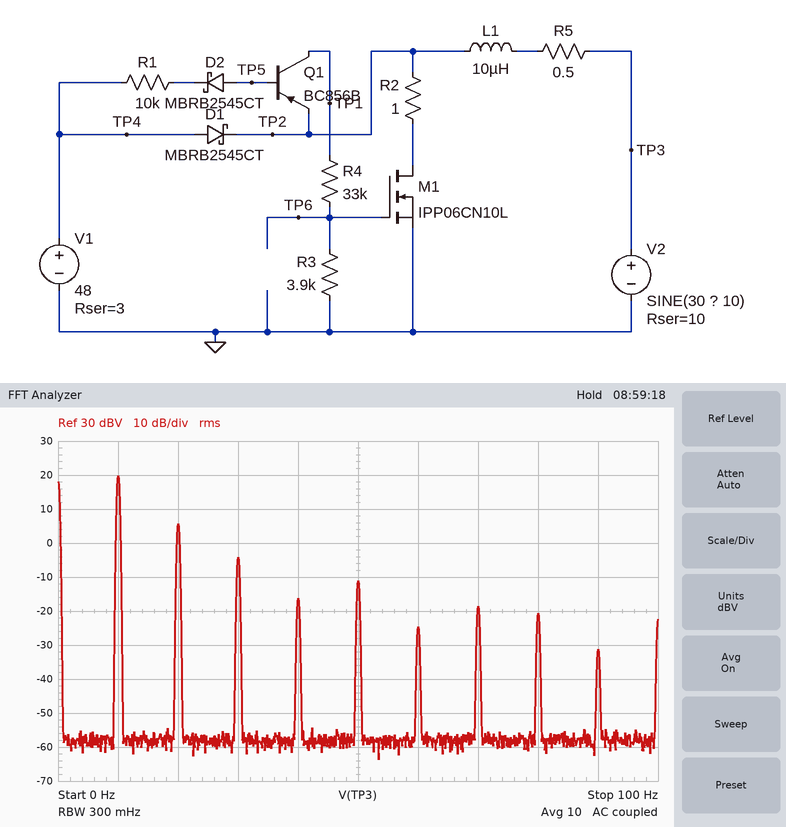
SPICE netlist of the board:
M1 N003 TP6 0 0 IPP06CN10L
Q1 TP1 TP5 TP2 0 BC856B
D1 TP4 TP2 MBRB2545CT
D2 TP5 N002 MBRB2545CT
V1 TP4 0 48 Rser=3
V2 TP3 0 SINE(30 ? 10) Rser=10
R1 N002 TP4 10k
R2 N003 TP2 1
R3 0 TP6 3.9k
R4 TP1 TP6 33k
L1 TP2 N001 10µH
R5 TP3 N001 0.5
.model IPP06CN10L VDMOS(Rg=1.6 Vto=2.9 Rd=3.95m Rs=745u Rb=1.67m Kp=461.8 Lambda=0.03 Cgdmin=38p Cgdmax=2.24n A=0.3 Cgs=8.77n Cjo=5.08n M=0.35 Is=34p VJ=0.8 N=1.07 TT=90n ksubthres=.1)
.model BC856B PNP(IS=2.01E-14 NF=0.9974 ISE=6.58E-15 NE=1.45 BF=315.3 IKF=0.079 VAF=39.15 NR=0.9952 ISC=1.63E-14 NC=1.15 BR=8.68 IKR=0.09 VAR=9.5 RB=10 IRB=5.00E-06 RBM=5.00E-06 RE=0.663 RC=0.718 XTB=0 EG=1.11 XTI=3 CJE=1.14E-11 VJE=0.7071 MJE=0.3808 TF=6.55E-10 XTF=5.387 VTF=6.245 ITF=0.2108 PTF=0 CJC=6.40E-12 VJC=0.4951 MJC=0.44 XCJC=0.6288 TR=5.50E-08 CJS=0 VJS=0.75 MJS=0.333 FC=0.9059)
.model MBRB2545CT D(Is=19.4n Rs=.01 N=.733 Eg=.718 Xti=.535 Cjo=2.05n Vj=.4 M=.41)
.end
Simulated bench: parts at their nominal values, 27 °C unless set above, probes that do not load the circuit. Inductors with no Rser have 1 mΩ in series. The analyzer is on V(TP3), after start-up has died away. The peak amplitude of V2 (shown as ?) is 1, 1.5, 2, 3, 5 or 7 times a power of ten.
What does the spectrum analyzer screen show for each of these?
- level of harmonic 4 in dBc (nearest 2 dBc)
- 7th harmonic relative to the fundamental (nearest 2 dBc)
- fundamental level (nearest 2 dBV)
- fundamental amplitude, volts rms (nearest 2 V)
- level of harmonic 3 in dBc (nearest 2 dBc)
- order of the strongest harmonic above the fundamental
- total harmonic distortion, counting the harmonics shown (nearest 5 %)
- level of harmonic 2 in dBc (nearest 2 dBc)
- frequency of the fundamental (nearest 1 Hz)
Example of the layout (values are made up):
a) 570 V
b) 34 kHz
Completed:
a) -36 dBc
b) -38 dBc
c) 20 dBV
d) 10 V
e) -24 dBc
f) 2
g) 20 %
h) -14 dBc
i) 10 Hz
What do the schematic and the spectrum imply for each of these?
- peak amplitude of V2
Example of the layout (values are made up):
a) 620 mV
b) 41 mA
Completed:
a) 70 V
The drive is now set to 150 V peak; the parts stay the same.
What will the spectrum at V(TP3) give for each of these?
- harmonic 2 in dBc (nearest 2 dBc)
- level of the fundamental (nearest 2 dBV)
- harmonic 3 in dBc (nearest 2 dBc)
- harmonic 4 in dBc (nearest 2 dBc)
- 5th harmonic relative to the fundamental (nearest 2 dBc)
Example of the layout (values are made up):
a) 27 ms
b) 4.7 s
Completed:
a) -12 dBc
b) 26 dBV
c) -28 dBc
d) -28 dBc
e) -34 dBc
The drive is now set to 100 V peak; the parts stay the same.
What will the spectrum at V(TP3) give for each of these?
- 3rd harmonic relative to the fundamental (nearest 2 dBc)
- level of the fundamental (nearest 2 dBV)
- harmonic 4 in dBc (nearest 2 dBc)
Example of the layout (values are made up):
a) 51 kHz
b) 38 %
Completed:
a) -26 dBc
b) 22 dBV
c) -30 dBc
